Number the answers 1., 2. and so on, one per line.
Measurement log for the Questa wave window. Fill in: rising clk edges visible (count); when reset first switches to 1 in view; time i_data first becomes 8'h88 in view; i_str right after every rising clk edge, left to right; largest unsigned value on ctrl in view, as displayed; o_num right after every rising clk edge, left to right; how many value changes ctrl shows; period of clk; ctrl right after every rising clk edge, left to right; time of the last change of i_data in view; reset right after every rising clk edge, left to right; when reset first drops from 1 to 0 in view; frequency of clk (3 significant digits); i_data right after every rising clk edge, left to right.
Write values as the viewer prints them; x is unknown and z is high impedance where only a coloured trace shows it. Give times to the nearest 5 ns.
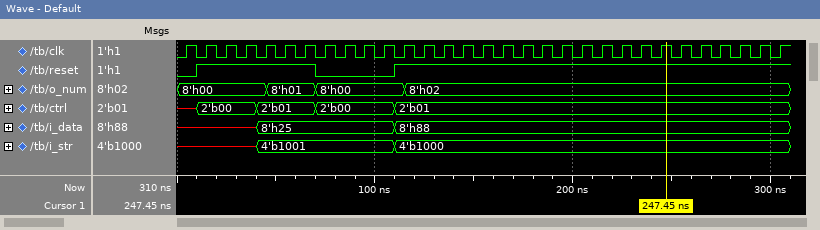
1. 31
2. 10 ns
3. 110 ns
4. x, x, x, x, 4'b1001, 4'b1001, 4'b1001, 4'b1001, 4'b1001, 4'b1001, 4'b1001, 4'b1000, 4'b1000, 4'b1000, 4'b1000, 4'b1000, 4'b1000, 4'b1000, 4'b1000, 4'b1000, 4'b1000, 4'b1000, 4'b1000, 4'b1000, 4'b1000, 4'b1000, 4'b1000, 4'b1000, 4'b1000, 4'b1000, 4'b1000
5. 2'b01
6. 8'h00, 8'h00, 8'h00, 8'h00, 8'h01, 8'h01, 8'h01, 8'h00, 8'h00, 8'h00, 8'h00, 8'h02, 8'h02, 8'h02, 8'h02, 8'h02, 8'h02, 8'h02, 8'h02, 8'h02, 8'h02, 8'h02, 8'h02, 8'h02, 8'h02, 8'h02, 8'h02, 8'h02, 8'h02, 8'h02, 8'h02
7. 4
8. 10 ns
9. x, 2'b00, 2'b00, 2'b00, 2'b01, 2'b01, 2'b01, 2'b00, 2'b00, 2'b00, 2'b00, 2'b01, 2'b01, 2'b01, 2'b01, 2'b01, 2'b01, 2'b01, 2'b01, 2'b01, 2'b01, 2'b01, 2'b01, 2'b01, 2'b01, 2'b01, 2'b01, 2'b01, 2'b01, 2'b01, 2'b01
10. 110 ns
11. 0 1 1 1 1 1 1 0 0 0 0 1 1 1 1 1 1 1 1 1 1 1 1 1 1 1 1 1 1 1 1
12. 70 ns
13. 100 MHz
14. x, x, x, x, 8'h25, 8'h25, 8'h25, 8'h25, 8'h25, 8'h25, 8'h25, 8'h88, 8'h88, 8'h88, 8'h88, 8'h88, 8'h88, 8'h88, 8'h88, 8'h88, 8'h88, 8'h88, 8'h88, 8'h88, 8'h88, 8'h88, 8'h88, 8'h88, 8'h88, 8'h88, 8'h88
